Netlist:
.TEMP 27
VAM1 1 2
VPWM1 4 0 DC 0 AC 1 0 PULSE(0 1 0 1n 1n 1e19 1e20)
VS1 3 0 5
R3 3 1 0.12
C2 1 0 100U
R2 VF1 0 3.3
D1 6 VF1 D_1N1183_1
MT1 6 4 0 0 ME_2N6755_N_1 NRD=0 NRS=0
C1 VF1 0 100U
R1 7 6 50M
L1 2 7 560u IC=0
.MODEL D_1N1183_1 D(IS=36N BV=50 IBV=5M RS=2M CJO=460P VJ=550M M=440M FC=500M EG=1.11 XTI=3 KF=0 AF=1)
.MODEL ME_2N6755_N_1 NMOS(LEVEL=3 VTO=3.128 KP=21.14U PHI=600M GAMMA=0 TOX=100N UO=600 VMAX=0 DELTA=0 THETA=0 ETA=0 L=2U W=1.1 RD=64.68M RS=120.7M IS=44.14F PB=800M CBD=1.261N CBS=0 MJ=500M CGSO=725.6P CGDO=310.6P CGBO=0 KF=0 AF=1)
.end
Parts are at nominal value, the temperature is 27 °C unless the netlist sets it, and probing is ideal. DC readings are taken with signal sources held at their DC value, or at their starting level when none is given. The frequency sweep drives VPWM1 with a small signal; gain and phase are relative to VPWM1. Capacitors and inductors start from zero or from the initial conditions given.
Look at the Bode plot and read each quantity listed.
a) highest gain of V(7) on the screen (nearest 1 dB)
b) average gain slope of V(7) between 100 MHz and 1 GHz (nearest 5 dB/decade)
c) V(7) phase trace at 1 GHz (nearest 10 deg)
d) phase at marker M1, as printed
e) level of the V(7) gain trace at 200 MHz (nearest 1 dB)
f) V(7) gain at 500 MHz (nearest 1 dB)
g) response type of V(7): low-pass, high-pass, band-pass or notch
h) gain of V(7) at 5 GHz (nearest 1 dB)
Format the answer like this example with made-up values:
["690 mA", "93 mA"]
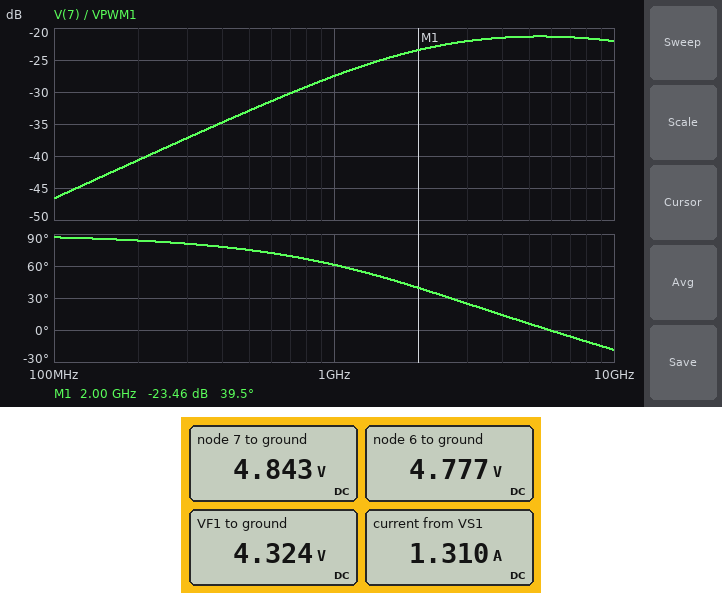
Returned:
["-21 dB", "20 dB/decade", "60 deg", "39.5 deg", "-41 dB", "-33 dB", "high-pass", "-21 dB"]
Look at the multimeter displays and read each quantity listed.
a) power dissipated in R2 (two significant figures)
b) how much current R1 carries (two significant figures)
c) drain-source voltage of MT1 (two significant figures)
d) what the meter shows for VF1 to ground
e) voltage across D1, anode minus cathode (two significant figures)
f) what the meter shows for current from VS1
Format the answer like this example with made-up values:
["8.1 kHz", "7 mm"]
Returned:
["5.7 W", "1.3 A", "4.8 V", "4.324 V", "450 mV", "1.310 A"]
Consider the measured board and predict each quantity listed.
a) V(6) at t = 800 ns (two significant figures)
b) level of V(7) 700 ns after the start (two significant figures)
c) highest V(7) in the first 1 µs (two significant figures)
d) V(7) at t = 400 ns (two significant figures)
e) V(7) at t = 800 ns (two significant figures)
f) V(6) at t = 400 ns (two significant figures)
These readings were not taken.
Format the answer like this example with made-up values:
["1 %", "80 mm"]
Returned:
["150 mV", "150 mV", "170 mV", "160 mV", "150 mV", "160 mV"]
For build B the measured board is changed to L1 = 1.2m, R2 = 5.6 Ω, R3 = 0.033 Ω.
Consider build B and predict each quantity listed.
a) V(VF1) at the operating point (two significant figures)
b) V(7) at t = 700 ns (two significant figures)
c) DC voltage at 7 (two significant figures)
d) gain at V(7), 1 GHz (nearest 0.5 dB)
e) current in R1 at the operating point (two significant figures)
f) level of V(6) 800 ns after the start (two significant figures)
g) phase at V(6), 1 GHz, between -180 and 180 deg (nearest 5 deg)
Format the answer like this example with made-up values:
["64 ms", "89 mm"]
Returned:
["4.5 V", "180 mV", "5.0 V", "-24.0 dB", "800 mA", "190 mV", "55 deg"]
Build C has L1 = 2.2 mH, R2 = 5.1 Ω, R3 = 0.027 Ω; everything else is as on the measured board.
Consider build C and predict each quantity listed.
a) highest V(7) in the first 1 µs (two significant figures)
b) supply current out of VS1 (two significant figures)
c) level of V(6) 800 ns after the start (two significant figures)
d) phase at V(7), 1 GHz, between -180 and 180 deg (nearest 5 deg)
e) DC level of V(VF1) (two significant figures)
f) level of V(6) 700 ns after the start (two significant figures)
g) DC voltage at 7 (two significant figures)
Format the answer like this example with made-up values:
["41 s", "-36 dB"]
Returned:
["200 mV", "880 mA", "180 mV", "55 deg", "4.5 V", "170 mV", "5.0 V"]
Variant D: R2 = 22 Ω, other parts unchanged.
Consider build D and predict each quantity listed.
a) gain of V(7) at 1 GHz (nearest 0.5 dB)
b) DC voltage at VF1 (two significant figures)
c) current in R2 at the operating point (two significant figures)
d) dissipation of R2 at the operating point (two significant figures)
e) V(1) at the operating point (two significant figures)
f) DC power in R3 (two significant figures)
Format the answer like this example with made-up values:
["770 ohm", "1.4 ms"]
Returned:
["-16.0 dB", "4.6 V", "210 mA", "950 mW", "5.0 V", "5.2 mW"]
